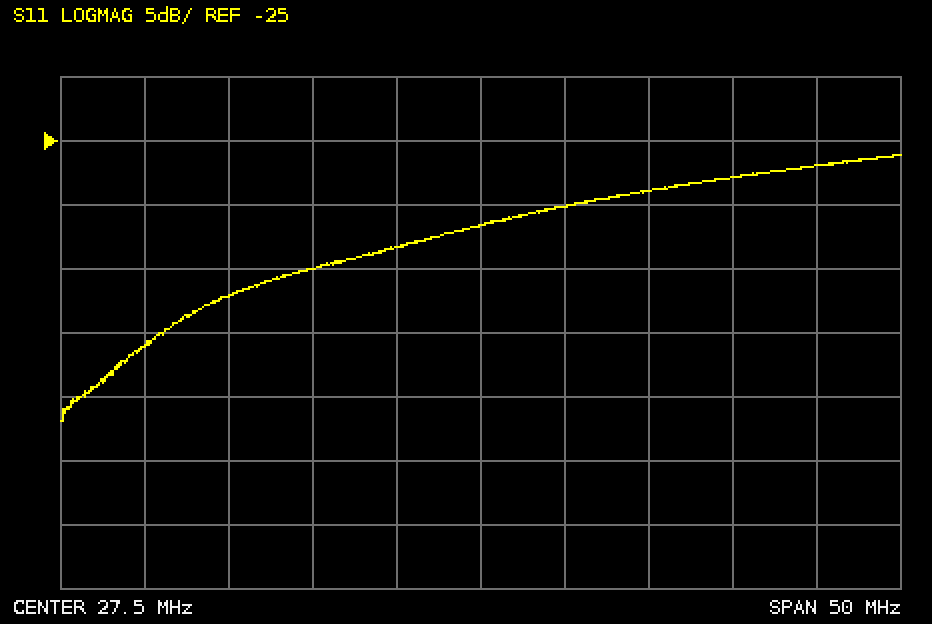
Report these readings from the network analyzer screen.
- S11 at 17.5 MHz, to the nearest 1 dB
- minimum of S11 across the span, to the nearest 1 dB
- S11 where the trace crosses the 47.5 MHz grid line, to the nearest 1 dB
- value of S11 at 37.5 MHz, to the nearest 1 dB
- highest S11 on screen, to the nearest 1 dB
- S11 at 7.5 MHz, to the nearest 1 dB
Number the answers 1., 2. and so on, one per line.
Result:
1. -35 dB
2. -47 dB
3. -27 dB
4. -29 dB
5. -26 dB
6. -41 dB
